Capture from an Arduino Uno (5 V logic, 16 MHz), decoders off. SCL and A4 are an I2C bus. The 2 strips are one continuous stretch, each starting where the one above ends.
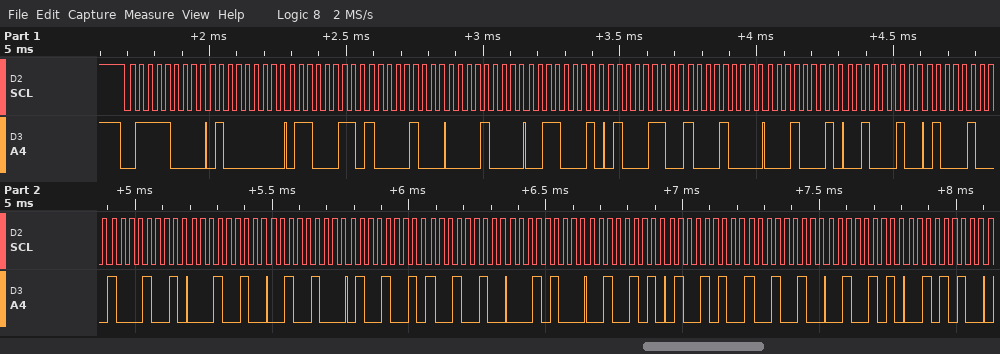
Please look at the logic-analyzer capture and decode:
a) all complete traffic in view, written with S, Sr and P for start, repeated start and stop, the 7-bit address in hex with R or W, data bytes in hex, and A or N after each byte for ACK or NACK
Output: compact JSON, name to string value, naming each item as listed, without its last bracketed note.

{"all complete traffic in view, written with S, Sr and P for start, repeated start and stop, the 7-bit address in hex with R or W, data bytes in hex, and A or N after each byte for ACK or NACK": "S 3CW A 40 A 63 A 84 A 08 A 31 A 46 A 88 A 11 A 22 A 44 A 89 A 12 A 24 A 49 A 92 A 14 A 25 A 4A A 92 A 25 A 2A A"}
